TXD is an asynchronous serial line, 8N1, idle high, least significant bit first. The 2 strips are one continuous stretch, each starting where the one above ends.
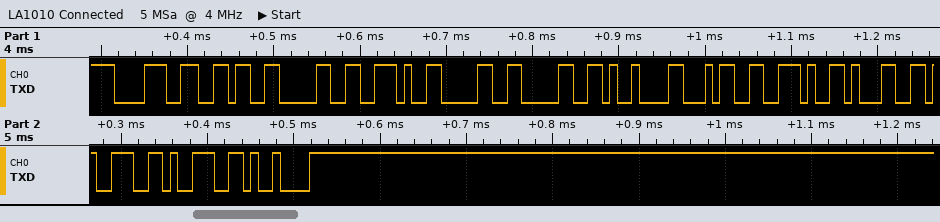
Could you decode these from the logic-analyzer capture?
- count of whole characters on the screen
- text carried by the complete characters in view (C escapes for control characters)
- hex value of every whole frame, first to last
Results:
13
"860.00\t4.199\t"
0x38 0x36 0x30 0x2E 0x30 0x30 0x09 0x34 0x2E 0x31 0x39 0x39 0x09
